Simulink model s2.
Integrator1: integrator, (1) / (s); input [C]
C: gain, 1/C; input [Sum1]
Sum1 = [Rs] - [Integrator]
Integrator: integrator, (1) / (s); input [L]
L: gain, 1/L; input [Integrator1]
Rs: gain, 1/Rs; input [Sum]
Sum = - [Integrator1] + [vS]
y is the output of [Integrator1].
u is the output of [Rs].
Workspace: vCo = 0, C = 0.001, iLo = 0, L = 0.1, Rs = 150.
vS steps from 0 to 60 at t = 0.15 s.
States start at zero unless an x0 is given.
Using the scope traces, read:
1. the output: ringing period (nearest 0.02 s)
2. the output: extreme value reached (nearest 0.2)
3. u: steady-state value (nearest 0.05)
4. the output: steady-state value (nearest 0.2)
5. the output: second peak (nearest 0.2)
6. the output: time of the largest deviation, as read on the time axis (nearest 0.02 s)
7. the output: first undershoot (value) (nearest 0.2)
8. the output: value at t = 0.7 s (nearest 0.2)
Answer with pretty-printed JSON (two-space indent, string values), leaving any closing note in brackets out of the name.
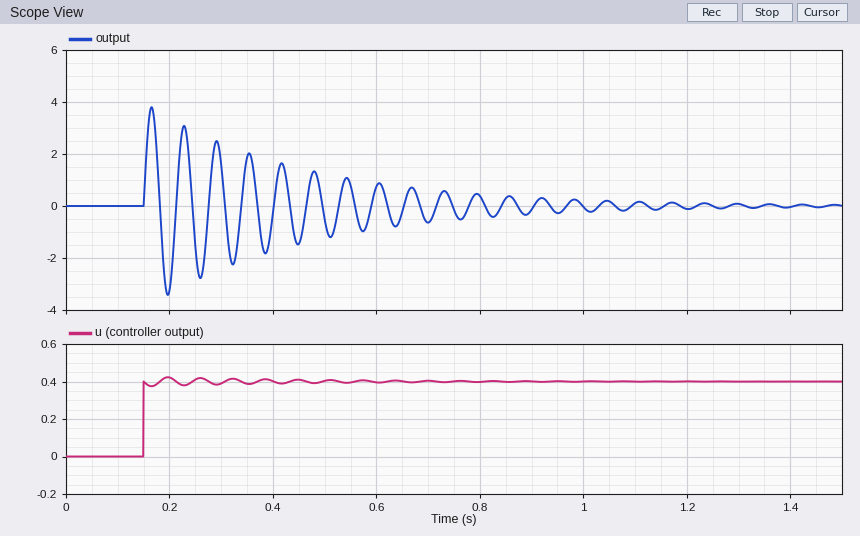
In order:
{
  "the output: ringing period": "0.06 s",
  "the output: extreme value reached": "3.8",
  "u: steady-state value": "0.40",
  "the output: steady-state value": "0.0",
  "the output: second peak": "3.0",
  "the output: time of the largest deviation, as read on the time axis": "0.16 s",
  "the output: first undershoot (value)": "-3.4",
  "the output: value at t = 0.7 s": "-0.6"
}
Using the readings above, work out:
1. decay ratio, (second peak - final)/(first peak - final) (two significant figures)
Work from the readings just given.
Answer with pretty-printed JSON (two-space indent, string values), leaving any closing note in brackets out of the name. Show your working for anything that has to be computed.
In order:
{
  "decay ratio, (second peak - final)/(first peak - final)": "(3 - 0) / (3.8 - 0) = 0.79"
}
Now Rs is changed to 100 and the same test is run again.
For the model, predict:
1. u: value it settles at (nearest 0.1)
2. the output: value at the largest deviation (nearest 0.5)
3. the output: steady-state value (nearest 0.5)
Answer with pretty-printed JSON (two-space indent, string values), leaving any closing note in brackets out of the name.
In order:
{
  "u: value it settles at": "0.6",
  "the output: value at the largest deviation": "5.5",
  "the output: steady-state value": "0.0"
}
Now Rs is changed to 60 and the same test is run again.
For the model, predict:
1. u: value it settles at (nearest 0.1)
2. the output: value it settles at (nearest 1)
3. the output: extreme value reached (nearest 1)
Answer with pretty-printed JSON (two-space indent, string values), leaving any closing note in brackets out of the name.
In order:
{
  "u: value it settles at": "1.0",
  "the output: value it settles at": "0",
  "the output: extreme value reached": "9"
}
